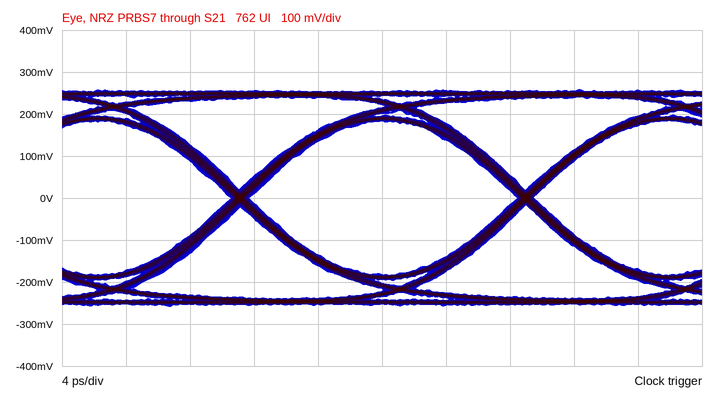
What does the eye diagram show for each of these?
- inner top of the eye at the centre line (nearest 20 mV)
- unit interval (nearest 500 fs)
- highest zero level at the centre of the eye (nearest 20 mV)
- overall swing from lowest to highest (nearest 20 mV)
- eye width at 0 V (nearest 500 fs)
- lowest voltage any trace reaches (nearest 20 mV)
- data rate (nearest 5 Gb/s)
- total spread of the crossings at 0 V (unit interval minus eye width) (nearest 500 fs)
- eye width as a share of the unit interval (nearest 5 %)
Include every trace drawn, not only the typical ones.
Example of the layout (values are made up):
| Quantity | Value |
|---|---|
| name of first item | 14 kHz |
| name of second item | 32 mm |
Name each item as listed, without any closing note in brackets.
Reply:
| Quantity | Value |
|---|---|
| inner top of the eye at the centre line | 180 mV |
| unit interval | 18.0 ps |
| highest zero level at the centre of the eye | -180 mV |
| overall swing from lowest to highest | 520 mV |
| eye width at 0 V | 17.0 ps |
| lowest voltage any trace reaches | -260 mV |
| data rate | 55 Gb/s |
| total spread of the crossings at 0 V (unit interval minus eye width) | 1.0 ps |
| eye width as a share of the unit interval | 95 % |
